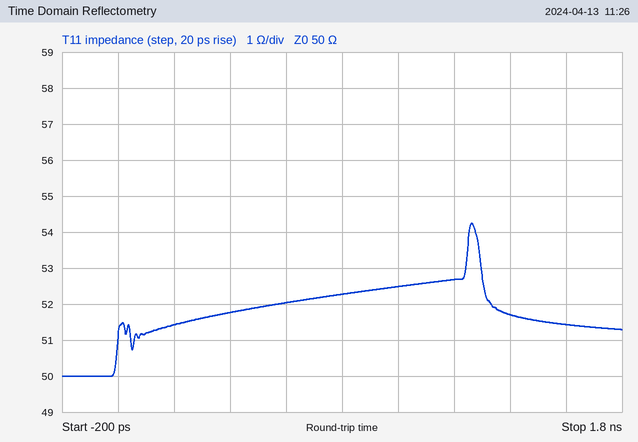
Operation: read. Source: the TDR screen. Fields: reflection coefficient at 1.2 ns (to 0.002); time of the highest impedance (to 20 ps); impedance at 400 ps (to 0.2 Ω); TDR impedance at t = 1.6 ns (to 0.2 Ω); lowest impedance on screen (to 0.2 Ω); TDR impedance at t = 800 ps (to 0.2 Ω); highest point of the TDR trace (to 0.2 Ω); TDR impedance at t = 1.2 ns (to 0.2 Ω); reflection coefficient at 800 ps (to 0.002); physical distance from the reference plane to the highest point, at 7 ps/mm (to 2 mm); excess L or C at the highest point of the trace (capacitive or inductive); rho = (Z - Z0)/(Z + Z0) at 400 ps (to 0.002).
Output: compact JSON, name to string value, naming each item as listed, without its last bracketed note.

{"reflection coefficient at 1.2 ns": "+0.026", "time of the highest impedance": "1.26 ns", "impedance at 400 ps": "51.8 Ω", "TDR impedance at t = 1.6 ns": "51.4 Ω", "lowest impedance on screen": "50.0 Ω", "TDR impedance at t = 800 ps": "52.2 Ω", "highest point of the TDR trace": "54.2 Ω", "TDR impedance at t = 1.2 ns": "52.6 Ω", "reflection coefficient at 800 ps": "+0.022", "physical distance from the reference plane to the highest point, at 7 ps/mm": "90 mm", "excess L or C at the highest point of the trace": "inductive", "rho = (Z - Z0)/(Z + Z0) at 400 ps": "+0.018"}
